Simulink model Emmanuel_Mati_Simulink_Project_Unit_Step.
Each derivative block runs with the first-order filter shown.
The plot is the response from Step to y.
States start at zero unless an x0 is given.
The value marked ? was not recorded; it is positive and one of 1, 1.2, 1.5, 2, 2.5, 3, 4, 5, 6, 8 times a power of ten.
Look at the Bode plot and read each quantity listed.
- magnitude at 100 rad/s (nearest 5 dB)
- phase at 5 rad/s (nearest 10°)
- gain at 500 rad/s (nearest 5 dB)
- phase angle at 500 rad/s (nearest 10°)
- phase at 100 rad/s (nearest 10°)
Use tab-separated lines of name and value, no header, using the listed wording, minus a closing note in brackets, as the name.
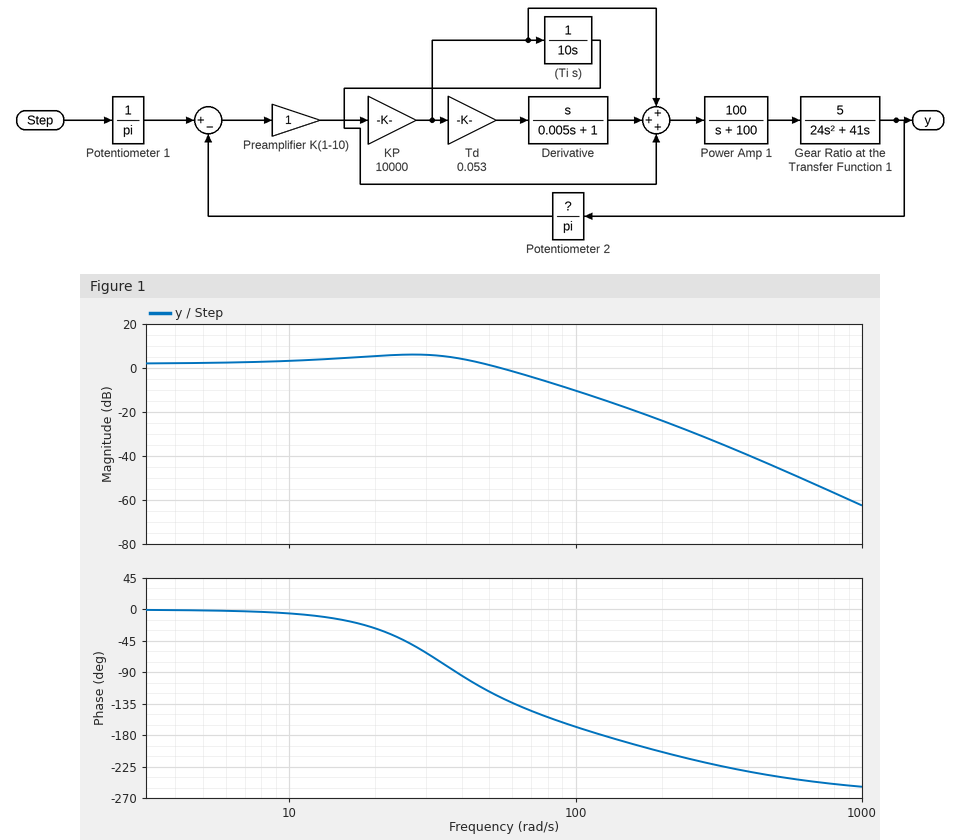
magnitude at 100 rad/s	-10 dB
phase at 5 rad/s	0°
gain at 500 rad/s	-45 dB
phase angle at 500 rad/s	-240°
phase at 100 rad/s	-170°
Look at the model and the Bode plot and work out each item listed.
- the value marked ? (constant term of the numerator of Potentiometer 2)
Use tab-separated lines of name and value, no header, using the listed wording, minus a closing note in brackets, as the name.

the value marked ?	0.8
